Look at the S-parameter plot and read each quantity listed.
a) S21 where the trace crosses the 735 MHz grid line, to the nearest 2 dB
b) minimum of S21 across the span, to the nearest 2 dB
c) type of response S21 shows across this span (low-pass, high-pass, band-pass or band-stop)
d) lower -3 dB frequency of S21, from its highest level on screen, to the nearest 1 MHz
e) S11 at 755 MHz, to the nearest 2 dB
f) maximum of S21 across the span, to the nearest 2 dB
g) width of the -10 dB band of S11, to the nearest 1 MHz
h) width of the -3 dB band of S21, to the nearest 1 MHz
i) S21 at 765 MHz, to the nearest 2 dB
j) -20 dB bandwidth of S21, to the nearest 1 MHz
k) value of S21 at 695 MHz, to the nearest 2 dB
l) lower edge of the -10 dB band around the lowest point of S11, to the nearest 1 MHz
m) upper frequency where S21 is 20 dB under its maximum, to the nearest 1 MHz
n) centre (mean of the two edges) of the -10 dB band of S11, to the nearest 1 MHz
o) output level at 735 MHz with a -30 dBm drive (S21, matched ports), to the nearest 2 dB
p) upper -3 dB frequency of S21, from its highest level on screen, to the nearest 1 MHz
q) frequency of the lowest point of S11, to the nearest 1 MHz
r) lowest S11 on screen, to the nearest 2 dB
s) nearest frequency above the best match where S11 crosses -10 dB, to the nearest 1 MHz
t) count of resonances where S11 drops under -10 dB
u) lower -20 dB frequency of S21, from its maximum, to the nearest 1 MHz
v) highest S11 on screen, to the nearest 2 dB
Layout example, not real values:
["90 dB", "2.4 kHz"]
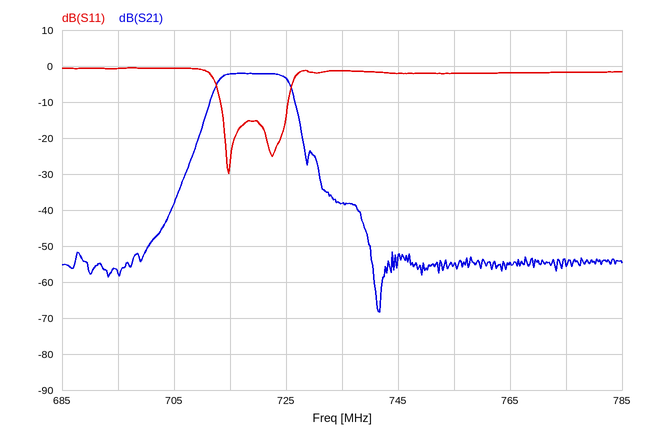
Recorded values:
["-38 dB", "-68 dB", "band-pass", "713 MHz", "-2 dB", "-2 dB", "12 MHz", "13 MHz", "-54 dB", "19 MHz", "-58 dB", "713 MHz", "728 MHz", "719 MHz", "-68 dBm", "726 MHz", "715 MHz", "-30 dB", "725 MHz", "2", "709 MHz", "0 dB"]
